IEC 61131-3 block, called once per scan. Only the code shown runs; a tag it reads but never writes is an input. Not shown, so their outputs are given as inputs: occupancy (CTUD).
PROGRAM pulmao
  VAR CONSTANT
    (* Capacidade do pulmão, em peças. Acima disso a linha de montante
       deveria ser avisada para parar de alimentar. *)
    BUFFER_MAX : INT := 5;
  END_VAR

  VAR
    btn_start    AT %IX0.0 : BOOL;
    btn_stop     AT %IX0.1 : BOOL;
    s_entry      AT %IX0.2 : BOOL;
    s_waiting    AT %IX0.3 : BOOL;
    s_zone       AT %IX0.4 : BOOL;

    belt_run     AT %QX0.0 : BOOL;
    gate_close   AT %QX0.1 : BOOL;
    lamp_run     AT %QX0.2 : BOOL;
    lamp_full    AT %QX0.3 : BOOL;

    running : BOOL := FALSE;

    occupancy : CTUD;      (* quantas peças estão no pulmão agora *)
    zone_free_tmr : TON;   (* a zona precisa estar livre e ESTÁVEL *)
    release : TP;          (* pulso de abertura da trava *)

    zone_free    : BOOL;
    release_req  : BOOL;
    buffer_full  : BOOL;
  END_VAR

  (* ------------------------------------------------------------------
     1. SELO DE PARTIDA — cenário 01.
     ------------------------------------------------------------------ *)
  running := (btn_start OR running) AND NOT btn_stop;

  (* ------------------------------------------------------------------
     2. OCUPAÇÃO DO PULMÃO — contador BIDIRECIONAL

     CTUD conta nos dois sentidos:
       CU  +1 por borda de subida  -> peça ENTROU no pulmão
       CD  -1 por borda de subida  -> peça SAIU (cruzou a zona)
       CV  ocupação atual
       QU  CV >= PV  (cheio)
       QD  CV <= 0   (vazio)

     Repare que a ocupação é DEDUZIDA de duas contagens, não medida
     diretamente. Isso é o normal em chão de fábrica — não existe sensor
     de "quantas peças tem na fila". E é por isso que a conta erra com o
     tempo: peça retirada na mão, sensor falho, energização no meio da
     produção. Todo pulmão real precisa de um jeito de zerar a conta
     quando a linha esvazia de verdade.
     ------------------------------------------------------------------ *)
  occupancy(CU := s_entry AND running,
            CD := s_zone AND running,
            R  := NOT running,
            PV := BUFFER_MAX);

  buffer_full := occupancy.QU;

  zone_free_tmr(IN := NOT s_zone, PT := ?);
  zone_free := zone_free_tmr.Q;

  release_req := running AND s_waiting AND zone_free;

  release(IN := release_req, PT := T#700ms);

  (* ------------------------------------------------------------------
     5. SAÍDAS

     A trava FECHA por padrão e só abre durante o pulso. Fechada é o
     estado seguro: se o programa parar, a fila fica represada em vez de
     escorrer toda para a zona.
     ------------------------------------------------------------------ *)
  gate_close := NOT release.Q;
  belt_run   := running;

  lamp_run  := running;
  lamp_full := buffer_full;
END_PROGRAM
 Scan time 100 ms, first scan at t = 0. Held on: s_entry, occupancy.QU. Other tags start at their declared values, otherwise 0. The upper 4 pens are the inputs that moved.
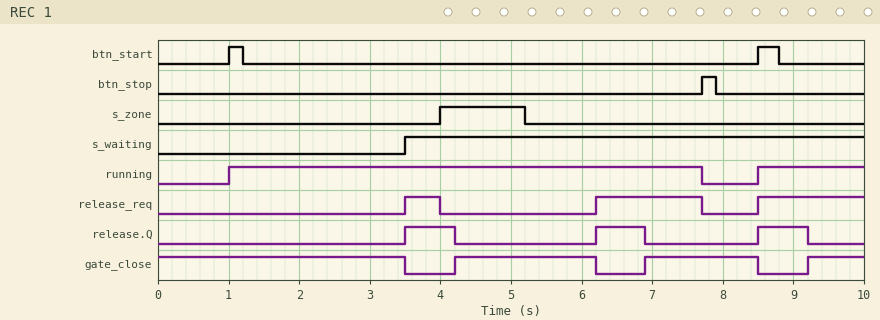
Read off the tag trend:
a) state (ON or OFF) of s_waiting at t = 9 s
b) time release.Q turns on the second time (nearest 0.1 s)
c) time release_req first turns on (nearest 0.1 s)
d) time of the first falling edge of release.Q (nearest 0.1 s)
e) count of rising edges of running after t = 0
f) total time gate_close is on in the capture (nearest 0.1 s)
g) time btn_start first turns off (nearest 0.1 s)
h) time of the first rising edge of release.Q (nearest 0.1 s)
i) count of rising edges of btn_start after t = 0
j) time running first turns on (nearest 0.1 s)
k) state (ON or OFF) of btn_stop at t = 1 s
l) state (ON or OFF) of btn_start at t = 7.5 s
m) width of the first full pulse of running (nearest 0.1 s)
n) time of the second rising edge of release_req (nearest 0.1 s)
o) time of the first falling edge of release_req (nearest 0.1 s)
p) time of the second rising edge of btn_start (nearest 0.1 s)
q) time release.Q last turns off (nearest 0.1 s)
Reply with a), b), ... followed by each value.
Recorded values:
a) ON
b) 6.2 s
c) 3.5 s
d) 4.2 s
e) 2
f) 7.9 s
g) 1.2 s
h) 3.5 s
i) 2
j) 1.0 s
k) OFF
l) OFF
m) 6.7 s
n) 6.2 s
o) 4.0 s
p) 8.5 s
q) 9.2 s
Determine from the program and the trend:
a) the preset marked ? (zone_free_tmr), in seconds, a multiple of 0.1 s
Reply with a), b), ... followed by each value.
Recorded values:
a) 1.0 s
